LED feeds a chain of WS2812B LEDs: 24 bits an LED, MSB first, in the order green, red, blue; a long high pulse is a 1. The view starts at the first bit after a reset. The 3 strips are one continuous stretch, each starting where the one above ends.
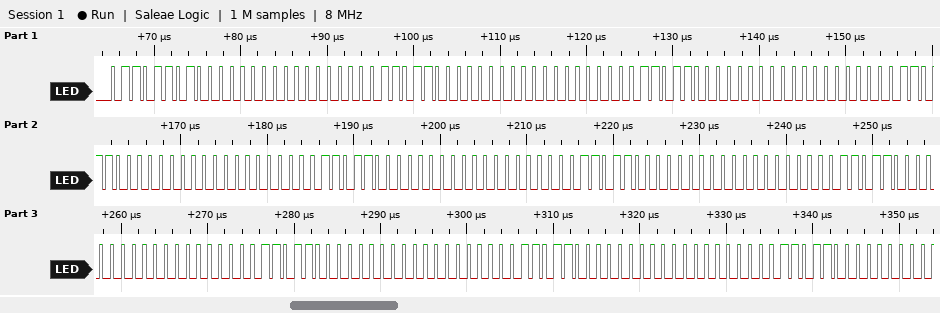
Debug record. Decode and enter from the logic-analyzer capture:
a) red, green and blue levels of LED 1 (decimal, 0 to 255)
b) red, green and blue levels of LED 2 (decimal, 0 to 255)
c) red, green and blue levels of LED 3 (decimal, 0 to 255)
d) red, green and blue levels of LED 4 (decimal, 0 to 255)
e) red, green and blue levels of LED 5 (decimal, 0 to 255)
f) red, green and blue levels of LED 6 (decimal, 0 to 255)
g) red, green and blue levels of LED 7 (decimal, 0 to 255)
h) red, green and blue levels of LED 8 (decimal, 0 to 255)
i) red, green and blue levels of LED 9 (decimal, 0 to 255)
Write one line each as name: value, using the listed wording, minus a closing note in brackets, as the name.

red, green and blue levels of LED 1: 0, 109, 0
red, green and blue levels of LED 2: 0, 108, 0
red, green and blue levels of LED 3: 0, 108, 0
red, green and blue levels of LED 4: 0, 108, 0
red, green and blue levels of LED 5: 0, 108, 0
red, green and blue levels of LED 6: 0, 108, 0
red, green and blue levels of LED 7: 0, 108, 0
red, green and blue levels of LED 8: 0, 108, 0
red, green and blue levels of LED 9: 0, 108, 0
